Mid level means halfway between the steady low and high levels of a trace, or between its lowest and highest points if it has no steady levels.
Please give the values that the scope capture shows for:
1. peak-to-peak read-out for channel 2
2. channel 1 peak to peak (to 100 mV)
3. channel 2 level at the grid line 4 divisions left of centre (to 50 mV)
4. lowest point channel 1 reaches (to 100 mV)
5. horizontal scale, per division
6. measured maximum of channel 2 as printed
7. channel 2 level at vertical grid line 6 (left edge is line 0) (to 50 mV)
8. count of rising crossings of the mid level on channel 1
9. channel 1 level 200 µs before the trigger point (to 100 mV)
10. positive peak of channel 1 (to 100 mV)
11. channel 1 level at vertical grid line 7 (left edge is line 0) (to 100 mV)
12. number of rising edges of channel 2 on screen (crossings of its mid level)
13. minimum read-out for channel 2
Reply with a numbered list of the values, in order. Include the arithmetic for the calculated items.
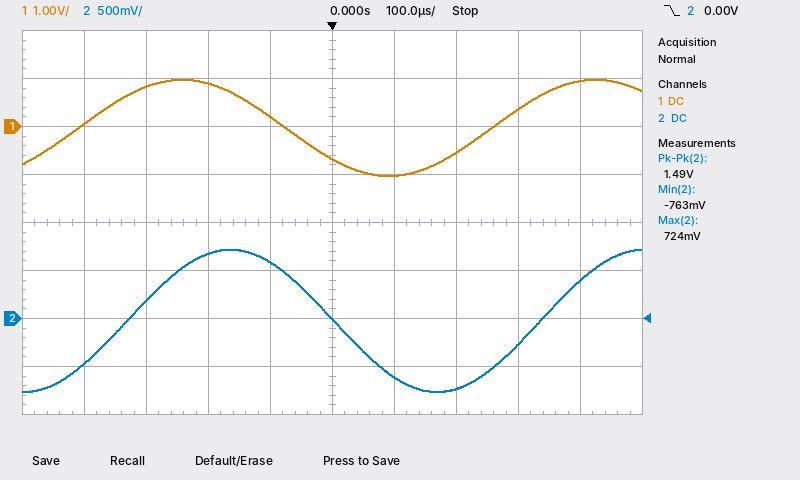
1. 1.49 V
2. 1.0 V − (-1.0 V) = 2.0 V
3. -450 mV
4. -1.0 V
5. 100 µs
6. 724 mV
7. -600 mV
8. 2
9. 900 mV
10. 1.0 V
11. -500 mV
12. 2
13. -763 mV
